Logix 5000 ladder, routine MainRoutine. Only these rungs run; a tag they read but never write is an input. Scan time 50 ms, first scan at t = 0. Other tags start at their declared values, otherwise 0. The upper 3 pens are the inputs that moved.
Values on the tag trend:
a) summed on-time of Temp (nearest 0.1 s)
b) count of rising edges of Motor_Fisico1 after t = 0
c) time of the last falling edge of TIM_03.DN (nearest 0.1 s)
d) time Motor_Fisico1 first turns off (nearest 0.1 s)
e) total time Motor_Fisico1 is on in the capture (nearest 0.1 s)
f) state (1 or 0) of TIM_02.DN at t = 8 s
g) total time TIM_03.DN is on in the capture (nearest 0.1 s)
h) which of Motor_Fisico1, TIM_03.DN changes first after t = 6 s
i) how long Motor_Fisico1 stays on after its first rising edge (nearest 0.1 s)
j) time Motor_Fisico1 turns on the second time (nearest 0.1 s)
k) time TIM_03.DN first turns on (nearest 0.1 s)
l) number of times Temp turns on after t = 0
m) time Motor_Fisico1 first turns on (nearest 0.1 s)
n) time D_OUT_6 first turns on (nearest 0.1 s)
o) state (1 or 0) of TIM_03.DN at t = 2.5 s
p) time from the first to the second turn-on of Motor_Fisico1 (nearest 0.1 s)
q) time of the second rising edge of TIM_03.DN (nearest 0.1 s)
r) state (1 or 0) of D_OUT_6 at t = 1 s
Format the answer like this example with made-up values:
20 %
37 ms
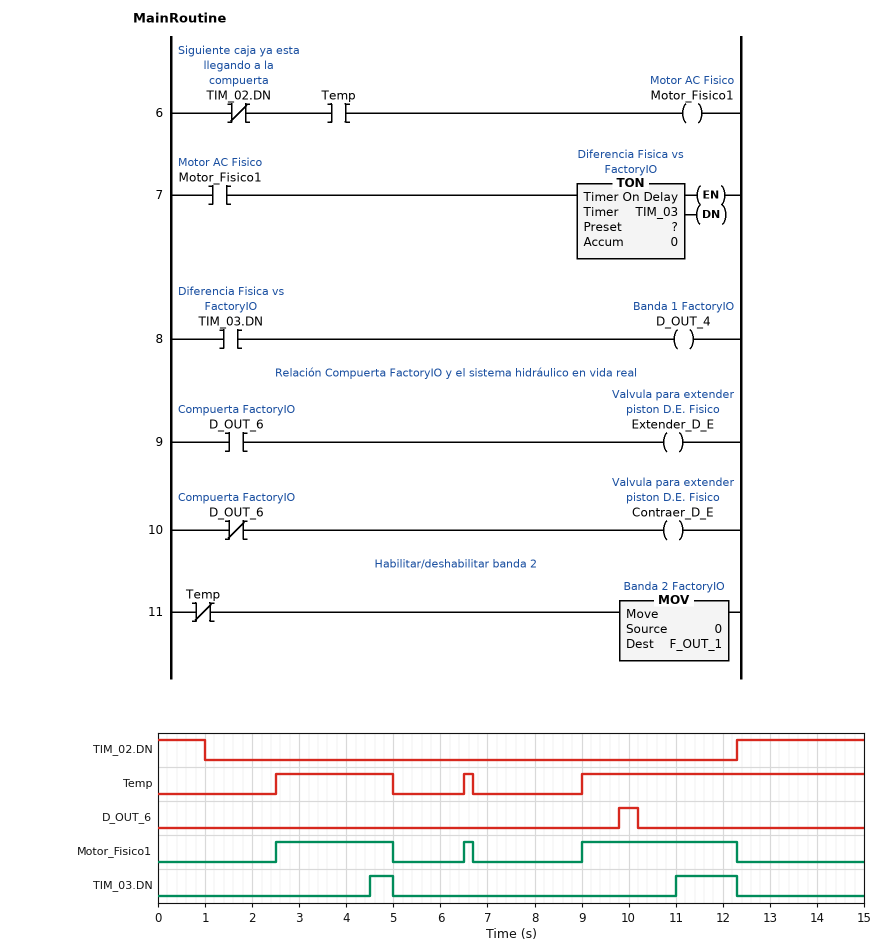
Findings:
8.7 s
3
12.3 s
5.0 s
6.0 s
0
1.8 s
Motor_Fisico1
2.5 s
6.5 s
4.5 s
3
2.5 s
9.8 s
0
4.0 s
11.0 s
0
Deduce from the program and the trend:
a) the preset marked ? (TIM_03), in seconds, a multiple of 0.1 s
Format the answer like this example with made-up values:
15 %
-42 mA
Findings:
2.0 s
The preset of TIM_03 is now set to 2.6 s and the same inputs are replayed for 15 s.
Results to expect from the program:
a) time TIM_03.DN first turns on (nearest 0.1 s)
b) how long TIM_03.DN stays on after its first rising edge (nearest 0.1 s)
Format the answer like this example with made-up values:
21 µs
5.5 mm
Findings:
11.6 s
0.7 s
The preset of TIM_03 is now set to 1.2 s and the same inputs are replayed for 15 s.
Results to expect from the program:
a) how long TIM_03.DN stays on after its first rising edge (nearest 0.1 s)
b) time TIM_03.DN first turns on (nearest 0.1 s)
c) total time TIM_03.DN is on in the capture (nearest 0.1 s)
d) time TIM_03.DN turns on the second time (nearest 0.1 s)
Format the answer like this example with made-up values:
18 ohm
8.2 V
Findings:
1.3 s
3.7 s
3.4 s
10.2 s
